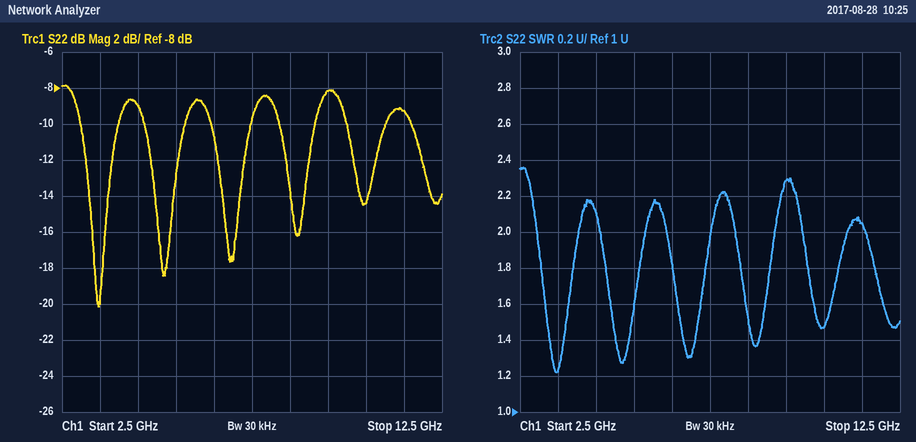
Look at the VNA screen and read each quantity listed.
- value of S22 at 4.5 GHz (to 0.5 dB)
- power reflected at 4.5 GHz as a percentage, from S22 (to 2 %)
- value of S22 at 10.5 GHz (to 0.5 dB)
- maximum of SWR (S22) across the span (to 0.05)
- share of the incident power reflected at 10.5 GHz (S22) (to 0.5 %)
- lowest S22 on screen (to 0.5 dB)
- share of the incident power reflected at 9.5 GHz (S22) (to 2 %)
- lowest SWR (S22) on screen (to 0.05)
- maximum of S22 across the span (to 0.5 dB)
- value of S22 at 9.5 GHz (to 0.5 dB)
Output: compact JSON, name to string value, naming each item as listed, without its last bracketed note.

{"value of S22 at 4.5 GHz": "-9.0 dB", "power reflected at 4.5 GHz as a percentage, from S22": "12 %", "value of S22 at 10.5 GHz": "-14.5 dB", "maximum of SWR (S22) across the span": "2.35", "share of the incident power reflected at 10.5 GHz (S22)": "3.5 %", "lowest S22 on screen": "-20.0 dB", "share of the incident power reflected at 9.5 GHz (S22)": "16 %", "lowest SWR (S22) on screen": "1.20", "maximum of S22 across the span": "-8.0 dB", "value of S22 at 9.5 GHz": "-8.0 dB"}
